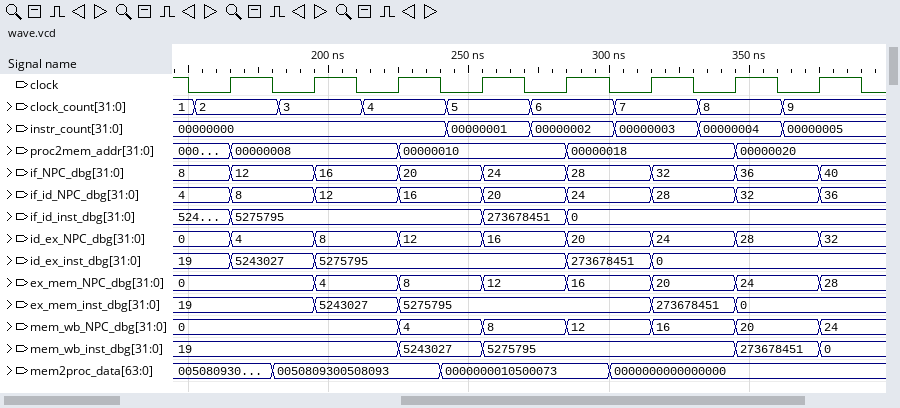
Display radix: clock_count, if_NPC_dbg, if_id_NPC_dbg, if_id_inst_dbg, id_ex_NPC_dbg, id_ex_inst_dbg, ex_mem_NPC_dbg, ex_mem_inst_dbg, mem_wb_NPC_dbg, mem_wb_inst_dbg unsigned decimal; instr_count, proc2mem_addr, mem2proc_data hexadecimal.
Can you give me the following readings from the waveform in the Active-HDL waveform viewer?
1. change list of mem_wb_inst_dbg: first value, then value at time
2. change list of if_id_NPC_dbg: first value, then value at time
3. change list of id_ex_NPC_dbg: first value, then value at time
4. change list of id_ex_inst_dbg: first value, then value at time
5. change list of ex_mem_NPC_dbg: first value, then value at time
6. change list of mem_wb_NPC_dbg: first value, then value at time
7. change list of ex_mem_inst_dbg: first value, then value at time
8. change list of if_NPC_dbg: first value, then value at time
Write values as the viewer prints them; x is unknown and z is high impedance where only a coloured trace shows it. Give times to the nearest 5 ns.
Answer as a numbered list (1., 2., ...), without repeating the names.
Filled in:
1. 19, 5243027 at 225 ns, 5275795 at 255 ns, 273678451 at 345 ns, 0 at 375 ns
2. 4, 8 at 165 ns, 12 at 195 ns, 16 at 225 ns, 20 at 255 ns, 24 at 285 ns, 28 at 315 ns, 32 at 345 ns, 36 at 375 ns
3. 0, 4 at 165 ns, 8 at 195 ns, 12 at 225 ns, 16 at 255 ns, 20 at 285 ns, 24 at 315 ns, 28 at 345 ns, 32 at 375 ns
4. 19, 5243027 at 165 ns, 5275795 at 195 ns, 273678451 at 285 ns, 0 at 315 ns
5. 0, 4 at 195 ns, 8 at 225 ns, 12 at 255 ns, 16 at 285 ns, 20 at 315 ns, 24 at 345 ns, 28 at 375 ns
6. 0, 4 at 225 ns, 8 at 255 ns, 12 at 285 ns, 16 at 315 ns, 20 at 345 ns, 24 at 375 ns
7. 19, 5243027 at 195 ns, 5275795 at 225 ns, 273678451 at 315 ns, 0 at 345 ns
8. 8, 12 at 165 ns, 16 at 195 ns, 20 at 225 ns, 24 at 255 ns, 28 at 285 ns, 32 at 315 ns, 36 at 345 ns, 40 at 375 ns
